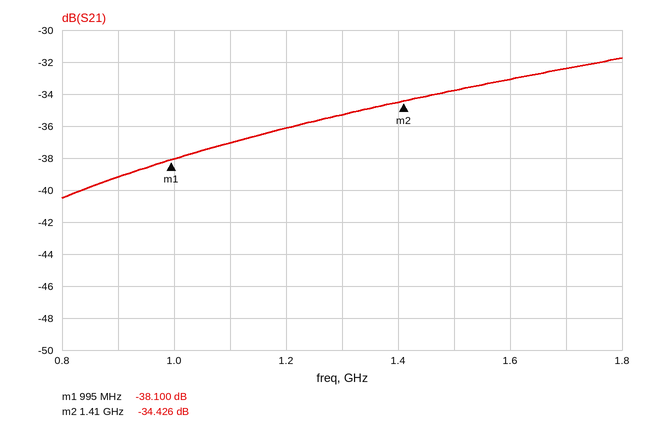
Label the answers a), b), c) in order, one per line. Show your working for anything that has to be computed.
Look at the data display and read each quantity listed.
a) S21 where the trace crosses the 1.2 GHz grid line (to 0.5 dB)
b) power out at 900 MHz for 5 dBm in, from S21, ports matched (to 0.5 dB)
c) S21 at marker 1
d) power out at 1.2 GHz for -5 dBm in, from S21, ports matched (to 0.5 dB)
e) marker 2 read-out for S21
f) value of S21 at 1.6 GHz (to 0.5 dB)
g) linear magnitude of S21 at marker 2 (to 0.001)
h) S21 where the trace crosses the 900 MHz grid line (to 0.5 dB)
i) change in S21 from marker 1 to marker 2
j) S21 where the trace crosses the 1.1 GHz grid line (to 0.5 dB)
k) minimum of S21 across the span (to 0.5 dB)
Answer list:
a) -36.0 dB
b) 5 dBm + (-39.0 dB) = -34.0 dBm
c) -38.100 dB
d) -5 dBm + (-36.0 dB) = -41.0 dBm
e) -34.426 dB
f) -33.0 dB
g) 10^(-34.426/20) ≈ 0.019
h) -39.0 dB
i) -34.426 − (-38.1) = 3.674 dB
j) -37.0 dB
k) -40.5 dB
